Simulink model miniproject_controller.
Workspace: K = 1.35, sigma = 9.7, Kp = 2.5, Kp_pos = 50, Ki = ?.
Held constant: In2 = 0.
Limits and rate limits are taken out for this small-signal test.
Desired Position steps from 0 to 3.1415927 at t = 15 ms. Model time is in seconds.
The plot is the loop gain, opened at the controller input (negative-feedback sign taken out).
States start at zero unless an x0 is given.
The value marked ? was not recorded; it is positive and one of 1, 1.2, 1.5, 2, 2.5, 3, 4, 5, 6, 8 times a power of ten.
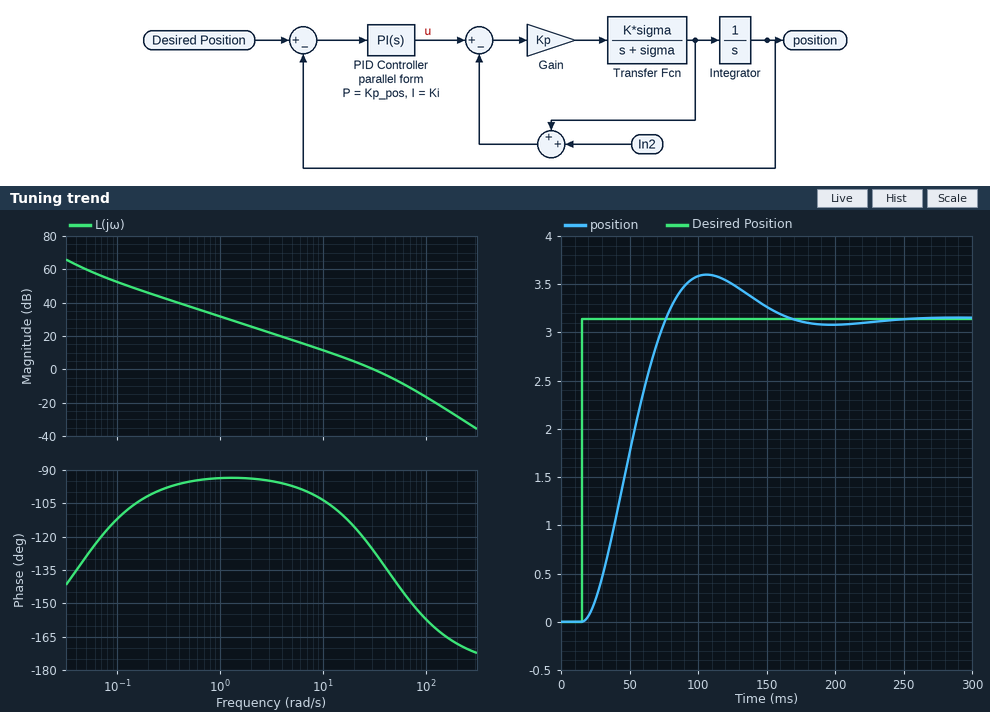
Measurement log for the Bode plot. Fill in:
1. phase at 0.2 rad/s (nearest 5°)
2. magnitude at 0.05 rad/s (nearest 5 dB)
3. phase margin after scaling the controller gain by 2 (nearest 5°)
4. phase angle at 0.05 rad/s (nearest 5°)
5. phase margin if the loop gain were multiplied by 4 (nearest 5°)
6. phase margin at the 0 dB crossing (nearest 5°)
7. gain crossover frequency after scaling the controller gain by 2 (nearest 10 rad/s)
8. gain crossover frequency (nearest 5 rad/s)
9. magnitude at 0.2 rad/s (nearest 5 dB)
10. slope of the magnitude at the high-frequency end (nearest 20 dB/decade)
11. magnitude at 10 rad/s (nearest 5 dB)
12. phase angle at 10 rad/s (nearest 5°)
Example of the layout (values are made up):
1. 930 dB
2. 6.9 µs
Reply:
1. -100°
2. 60 dB
3. 40°
4. -130°
5. 30°
6. 55°
7. 50 rad/s
8. 30 rad/s
9. 45 dB
10. -40 dB/decade
11. 10 dB
12. -105°
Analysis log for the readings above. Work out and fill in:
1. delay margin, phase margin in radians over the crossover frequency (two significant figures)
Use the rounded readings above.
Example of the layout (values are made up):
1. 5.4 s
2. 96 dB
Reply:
1. 0.032 s
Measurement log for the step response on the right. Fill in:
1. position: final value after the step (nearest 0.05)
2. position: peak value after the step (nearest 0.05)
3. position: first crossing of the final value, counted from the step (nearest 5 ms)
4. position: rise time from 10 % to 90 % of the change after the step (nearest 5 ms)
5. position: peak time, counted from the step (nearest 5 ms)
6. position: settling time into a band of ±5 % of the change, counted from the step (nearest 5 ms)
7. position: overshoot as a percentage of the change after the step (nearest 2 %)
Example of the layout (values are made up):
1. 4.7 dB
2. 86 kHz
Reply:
1. 3.15
2. 3.60
3. 60 ms
4. 40 ms
5. 90 ms
6. 130 ms
7. 14 %
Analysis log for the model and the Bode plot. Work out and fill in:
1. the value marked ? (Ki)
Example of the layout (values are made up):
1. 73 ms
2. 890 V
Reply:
1. 2
